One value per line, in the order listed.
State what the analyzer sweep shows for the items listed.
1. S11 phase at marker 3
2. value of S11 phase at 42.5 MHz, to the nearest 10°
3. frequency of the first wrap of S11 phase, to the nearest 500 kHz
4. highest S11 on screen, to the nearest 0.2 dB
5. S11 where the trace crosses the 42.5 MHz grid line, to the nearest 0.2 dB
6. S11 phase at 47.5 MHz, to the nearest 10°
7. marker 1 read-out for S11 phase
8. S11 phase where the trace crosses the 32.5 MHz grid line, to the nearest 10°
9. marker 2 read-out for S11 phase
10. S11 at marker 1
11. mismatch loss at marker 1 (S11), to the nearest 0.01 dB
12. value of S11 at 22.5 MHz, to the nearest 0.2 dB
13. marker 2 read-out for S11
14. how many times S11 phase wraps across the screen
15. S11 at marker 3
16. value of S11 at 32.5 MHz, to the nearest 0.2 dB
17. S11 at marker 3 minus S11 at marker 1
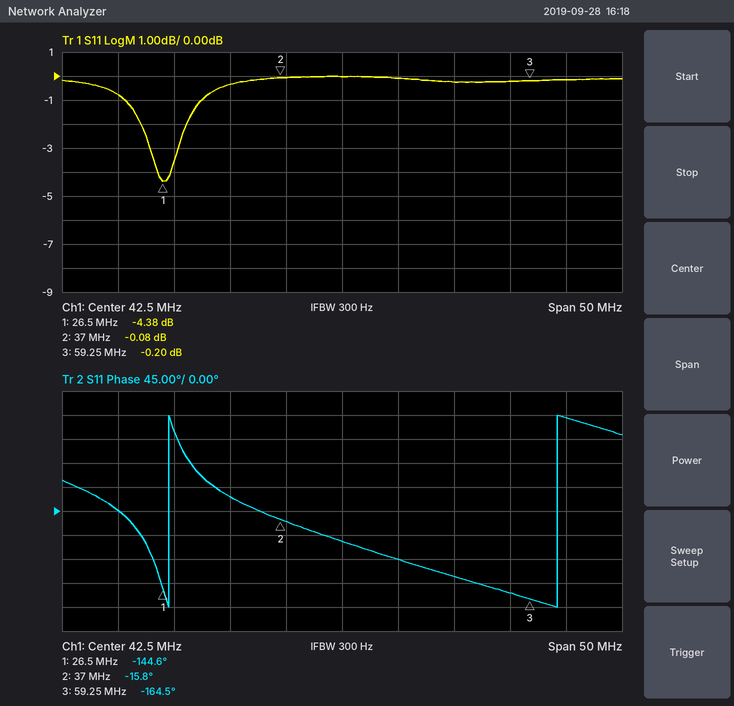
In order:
-164.5°
-60°
27.0 MHz
0.0 dB
0.0 dB
-90°
-144.6°
30°
-15.8°
-4.38 dB
1.97 dB
-0.8 dB
-0.08 dB
2
-0.20 dB
-0.4 dB
4.18 dB
